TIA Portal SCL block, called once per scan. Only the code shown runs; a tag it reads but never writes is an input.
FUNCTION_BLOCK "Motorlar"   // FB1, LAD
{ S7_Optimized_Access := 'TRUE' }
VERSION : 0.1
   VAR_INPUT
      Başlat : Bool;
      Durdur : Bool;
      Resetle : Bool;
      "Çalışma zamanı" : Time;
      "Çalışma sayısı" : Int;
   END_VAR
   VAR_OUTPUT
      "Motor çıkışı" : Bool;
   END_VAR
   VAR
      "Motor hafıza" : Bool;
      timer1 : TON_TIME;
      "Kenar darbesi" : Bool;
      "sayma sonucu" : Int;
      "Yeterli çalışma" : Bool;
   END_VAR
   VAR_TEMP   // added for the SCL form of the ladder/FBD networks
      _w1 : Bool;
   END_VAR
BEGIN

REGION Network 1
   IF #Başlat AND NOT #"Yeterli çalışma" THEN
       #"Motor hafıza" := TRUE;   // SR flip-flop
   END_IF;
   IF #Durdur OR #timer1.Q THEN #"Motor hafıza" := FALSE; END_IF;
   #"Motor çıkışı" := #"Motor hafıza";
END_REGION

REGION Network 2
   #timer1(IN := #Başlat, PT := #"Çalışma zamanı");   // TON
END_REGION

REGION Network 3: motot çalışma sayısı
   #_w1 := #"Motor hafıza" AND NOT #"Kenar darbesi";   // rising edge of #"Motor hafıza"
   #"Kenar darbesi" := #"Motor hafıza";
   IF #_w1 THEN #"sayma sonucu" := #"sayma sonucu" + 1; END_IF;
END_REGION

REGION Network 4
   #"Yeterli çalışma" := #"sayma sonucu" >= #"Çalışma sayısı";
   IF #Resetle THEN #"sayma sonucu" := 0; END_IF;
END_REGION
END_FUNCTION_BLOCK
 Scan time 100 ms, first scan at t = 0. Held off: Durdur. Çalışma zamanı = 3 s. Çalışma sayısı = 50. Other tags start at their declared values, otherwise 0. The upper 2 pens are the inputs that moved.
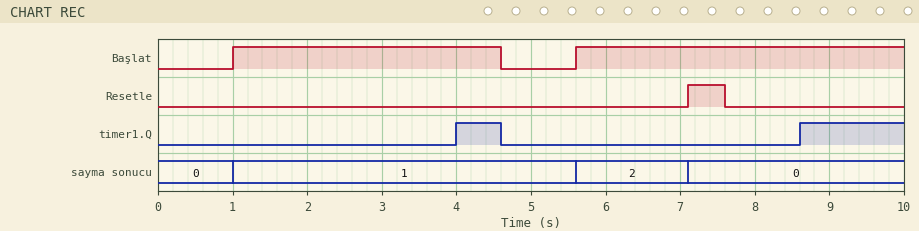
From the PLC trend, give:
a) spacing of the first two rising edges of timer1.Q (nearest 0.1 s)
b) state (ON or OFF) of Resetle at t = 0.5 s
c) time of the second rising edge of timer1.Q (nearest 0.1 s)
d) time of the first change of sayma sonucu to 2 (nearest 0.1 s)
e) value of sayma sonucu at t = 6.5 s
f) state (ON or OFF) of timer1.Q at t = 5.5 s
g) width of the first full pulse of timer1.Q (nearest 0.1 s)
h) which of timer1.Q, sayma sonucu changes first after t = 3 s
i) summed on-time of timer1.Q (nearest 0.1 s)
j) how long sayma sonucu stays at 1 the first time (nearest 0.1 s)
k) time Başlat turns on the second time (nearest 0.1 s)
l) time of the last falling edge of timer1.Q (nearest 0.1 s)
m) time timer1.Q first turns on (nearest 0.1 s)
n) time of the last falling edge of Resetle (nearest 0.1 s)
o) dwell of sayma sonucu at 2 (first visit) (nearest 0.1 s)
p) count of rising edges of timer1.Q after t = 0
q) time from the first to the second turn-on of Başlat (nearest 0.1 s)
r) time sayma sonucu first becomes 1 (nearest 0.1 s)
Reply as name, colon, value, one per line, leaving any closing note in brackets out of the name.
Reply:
spacing of the first two rising edges of timer1.Q: 4.6 s
state (ON or OFF) of Resetle at t = 0.5 s: OFF
time of the second rising edge of timer1.Q: 8.6 s
time of the first change of sayma sonucu to 2: 5.6 s
value of sayma sonucu at t = 6.5 s: 2
state (ON or OFF) of timer1.Q at t = 5.5 s: OFF
width of the first full pulse of timer1.Q: 0.6 s
which of timer1.Q, sayma sonucu changes first after t = 3 s: timer1.Q
summed on-time of timer1.Q: 2.0 s
how long sayma sonucu stays at 1 the first time: 4.6 s
time Başlat turns on the second time: 5.6 s
time of the last falling edge of timer1.Q: 4.6 s
time timer1.Q first turns on: 4.0 s
time of the last falling edge of Resetle: 7.6 s
dwell of sayma sonucu at 2 (first visit): 1.5 s
count of rising edges of timer1.Q after t = 0: 2
time from the first to the second turn-on of Başlat: 4.6 s
time sayma sonucu first becomes 1: 1.0 s
